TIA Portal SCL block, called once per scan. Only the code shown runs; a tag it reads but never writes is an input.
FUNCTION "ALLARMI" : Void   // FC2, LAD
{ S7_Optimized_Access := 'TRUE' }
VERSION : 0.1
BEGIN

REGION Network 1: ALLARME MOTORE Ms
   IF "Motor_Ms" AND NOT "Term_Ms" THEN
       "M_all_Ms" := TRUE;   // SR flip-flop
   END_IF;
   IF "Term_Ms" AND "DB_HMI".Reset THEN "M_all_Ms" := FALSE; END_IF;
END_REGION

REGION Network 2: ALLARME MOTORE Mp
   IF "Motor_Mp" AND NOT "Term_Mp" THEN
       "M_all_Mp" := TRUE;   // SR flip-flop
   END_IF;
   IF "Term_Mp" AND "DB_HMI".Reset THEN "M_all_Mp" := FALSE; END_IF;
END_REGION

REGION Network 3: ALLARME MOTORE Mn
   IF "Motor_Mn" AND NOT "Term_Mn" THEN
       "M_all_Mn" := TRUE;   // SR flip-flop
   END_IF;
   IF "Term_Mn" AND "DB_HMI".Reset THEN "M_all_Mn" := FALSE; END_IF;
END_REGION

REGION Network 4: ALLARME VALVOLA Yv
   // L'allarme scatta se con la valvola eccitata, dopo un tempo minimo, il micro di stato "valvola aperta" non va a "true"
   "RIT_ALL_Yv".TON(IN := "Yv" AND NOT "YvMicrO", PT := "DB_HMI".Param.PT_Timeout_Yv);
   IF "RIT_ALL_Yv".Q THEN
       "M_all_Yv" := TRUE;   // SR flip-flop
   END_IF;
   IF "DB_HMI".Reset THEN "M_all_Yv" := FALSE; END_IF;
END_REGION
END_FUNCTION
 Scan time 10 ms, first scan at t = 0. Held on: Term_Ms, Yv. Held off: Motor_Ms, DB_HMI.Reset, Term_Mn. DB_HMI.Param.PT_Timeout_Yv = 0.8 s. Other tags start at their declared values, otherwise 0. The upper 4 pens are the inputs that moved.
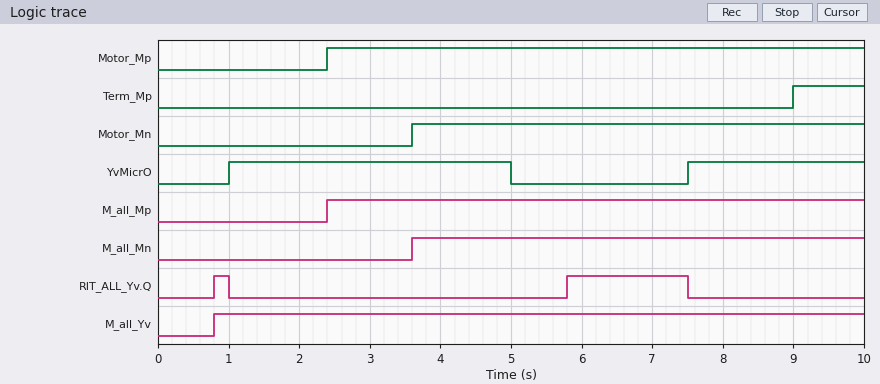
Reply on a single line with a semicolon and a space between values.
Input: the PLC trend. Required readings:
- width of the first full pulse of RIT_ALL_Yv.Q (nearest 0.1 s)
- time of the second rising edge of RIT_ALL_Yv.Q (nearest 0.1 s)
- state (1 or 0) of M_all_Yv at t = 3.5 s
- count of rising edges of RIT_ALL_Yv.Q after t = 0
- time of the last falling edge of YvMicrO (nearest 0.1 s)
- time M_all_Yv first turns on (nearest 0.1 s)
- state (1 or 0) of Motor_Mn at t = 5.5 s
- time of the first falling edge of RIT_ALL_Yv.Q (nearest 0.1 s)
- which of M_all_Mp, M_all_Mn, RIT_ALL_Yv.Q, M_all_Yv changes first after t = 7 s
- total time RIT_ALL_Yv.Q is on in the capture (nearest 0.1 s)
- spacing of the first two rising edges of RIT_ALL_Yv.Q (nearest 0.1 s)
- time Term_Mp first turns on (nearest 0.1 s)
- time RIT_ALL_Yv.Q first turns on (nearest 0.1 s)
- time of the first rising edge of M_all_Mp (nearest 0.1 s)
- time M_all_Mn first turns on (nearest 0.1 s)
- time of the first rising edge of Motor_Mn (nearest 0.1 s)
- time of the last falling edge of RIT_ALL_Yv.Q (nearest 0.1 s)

0.2 s; 5.8 s; 1; 2; 5.0 s; 0.8 s; 1; 1.0 s; RIT_ALL_Yv.Q; 1.9 s; 5.0 s; 9.0 s; 0.8 s; 2.4 s; 3.6 s; 3.6 s; 7.5 s
